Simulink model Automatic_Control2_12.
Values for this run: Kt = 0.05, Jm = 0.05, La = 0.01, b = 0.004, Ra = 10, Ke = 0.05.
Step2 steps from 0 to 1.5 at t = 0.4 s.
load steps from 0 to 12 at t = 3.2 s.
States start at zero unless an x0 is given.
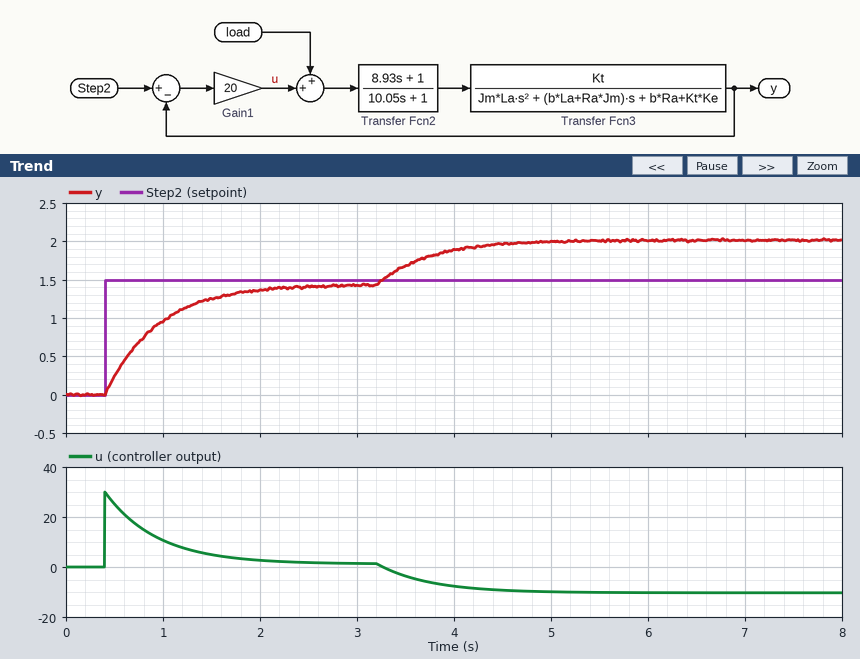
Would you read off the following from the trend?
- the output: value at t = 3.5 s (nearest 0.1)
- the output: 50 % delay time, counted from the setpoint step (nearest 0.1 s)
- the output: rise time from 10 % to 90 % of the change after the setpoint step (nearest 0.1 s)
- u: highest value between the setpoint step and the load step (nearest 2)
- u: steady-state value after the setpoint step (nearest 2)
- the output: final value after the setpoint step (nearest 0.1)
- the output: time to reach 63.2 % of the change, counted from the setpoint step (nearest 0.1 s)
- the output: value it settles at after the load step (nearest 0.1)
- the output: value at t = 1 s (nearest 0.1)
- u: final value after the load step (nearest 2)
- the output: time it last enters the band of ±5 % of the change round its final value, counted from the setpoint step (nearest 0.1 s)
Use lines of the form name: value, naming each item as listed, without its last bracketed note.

the output: value at t = 3.5 s: 1.7
the output: 50 % delay time, counted from the setpoint step: 0.4 s
the output: rise time from 10 % to 90 % of the change after the setpoint step: 1.2 s
u: highest value between the setpoint step and the load step: 30
u: steady-state value after the setpoint step: 2
the output: final value after the setpoint step: 1.4
the output: time to reach 63.2 % of the change, counted from the setpoint step: 0.5 s
the output: value it settles at after the load step: 2.0
the output: value at t = 1 s: 1.0
u: final value after the load step: -10
the output: time it last enters the band of ±5 % of the change round its final value, counted from the setpoint step: 1.6 s
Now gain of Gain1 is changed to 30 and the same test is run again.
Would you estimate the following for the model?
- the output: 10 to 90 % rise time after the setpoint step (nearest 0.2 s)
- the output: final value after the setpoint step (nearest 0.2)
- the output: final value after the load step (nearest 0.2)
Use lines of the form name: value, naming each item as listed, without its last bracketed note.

the output: 10 to 90 % rise time after the setpoint step: 0.8 s
the output: final value after the setpoint step: 1.4
the output: final value after the load step: 1.8
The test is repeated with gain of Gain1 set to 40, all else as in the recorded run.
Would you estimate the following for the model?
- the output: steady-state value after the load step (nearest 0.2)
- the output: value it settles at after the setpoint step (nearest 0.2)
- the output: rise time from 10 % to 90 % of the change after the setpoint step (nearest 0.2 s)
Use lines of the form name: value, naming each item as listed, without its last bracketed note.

the output: steady-state value after the load step: 1.8
the output: value it settles at after the setpoint step: 1.4
the output: rise time from 10 % to 90 % of the change after the setpoint step: 0.6 s
